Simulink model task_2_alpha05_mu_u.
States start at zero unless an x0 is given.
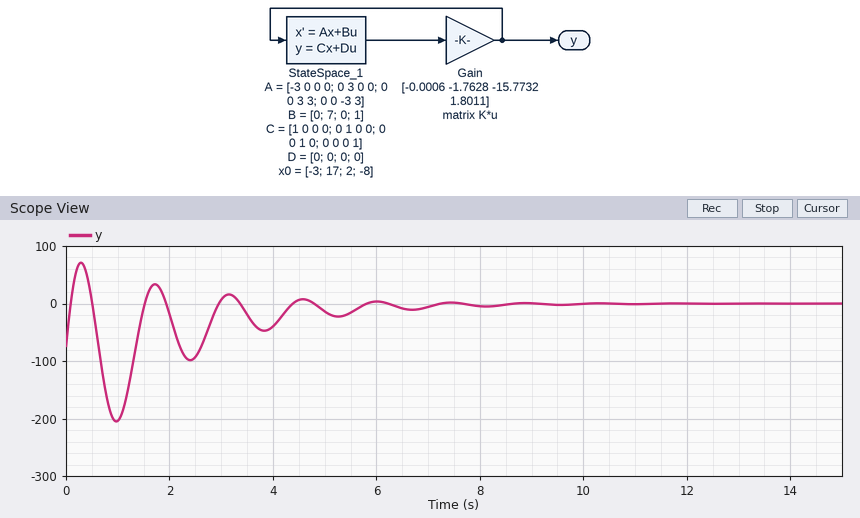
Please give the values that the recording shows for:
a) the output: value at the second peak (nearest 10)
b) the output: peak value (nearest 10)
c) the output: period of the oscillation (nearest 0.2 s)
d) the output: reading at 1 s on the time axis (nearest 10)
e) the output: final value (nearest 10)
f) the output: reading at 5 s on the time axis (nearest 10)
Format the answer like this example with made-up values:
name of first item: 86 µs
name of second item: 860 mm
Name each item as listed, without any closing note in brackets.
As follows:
the output: value at the second peak: 30
the output: peak value: 70
the output: period of the oscillation: 1.4 s
the output: reading at 1 s on the time axis: -200
the output: final value: 0
the output: reading at 5 s on the time axis: -10
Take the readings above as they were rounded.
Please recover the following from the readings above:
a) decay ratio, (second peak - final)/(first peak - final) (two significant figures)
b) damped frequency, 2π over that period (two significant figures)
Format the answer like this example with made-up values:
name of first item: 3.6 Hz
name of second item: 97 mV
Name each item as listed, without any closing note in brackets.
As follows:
decay ratio, (second peak - final)/(first peak - final): 0.43
damped frequency, 2π over that period: 4.5 rad/s
